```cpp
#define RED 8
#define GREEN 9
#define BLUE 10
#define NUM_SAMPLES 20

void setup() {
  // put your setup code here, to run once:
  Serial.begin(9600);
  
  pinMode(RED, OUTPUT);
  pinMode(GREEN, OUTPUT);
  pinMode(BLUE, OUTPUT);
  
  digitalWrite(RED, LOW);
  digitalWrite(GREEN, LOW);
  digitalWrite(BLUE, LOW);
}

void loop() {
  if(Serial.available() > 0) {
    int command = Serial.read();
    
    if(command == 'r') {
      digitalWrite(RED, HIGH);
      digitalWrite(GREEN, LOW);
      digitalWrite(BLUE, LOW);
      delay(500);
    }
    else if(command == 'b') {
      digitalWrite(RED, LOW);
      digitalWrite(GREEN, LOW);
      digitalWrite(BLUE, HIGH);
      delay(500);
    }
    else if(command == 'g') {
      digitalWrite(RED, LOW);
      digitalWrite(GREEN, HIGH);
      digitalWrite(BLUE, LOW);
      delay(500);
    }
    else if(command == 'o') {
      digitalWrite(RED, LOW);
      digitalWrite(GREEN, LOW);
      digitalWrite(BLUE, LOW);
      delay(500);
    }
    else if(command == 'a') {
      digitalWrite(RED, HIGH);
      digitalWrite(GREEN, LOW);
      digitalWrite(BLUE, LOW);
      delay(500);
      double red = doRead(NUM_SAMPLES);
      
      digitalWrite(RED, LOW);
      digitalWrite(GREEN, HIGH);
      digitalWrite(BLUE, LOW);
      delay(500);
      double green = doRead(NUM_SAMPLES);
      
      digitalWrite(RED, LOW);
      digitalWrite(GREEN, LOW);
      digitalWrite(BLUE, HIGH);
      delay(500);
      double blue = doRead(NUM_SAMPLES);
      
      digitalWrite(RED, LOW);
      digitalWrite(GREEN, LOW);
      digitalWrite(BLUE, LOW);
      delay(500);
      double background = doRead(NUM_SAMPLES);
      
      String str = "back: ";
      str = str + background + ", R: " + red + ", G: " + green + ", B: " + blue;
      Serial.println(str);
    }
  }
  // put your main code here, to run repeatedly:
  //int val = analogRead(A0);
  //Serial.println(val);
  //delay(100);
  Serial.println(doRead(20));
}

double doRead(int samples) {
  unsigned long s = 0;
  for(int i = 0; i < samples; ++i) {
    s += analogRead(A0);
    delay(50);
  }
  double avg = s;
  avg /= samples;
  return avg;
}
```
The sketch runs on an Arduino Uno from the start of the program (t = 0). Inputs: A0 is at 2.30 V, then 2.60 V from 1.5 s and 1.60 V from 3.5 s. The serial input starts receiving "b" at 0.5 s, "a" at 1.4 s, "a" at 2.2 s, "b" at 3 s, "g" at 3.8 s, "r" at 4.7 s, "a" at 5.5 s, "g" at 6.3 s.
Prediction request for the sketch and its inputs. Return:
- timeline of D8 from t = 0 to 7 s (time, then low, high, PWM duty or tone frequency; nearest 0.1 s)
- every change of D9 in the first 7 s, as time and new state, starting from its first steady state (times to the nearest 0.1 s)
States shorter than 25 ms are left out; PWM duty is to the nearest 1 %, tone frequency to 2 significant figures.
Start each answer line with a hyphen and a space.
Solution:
- 0 s low; 2.5 s high; 4 s low
- 0 s low; 4 s high; 5.5 s low
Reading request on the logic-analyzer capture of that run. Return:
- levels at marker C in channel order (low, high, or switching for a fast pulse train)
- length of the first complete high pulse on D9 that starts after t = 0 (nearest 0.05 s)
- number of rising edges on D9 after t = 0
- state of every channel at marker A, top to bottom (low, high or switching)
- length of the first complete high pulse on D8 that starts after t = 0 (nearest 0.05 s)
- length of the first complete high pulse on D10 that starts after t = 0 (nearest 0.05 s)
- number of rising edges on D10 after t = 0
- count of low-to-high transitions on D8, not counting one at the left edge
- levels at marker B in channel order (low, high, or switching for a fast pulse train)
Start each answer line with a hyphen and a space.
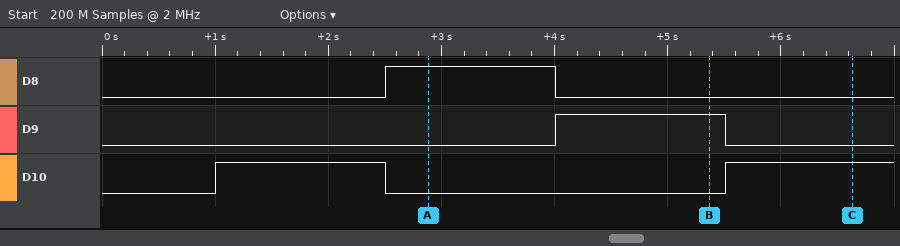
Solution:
- D8 low, D9 low, D10 high
- 1.50 s
- 1
- D8 high, D9 low, D10 low
- 1.50 s
- 1.50 s
- 2
- 1
- D8 low, D9 high, D10 low
